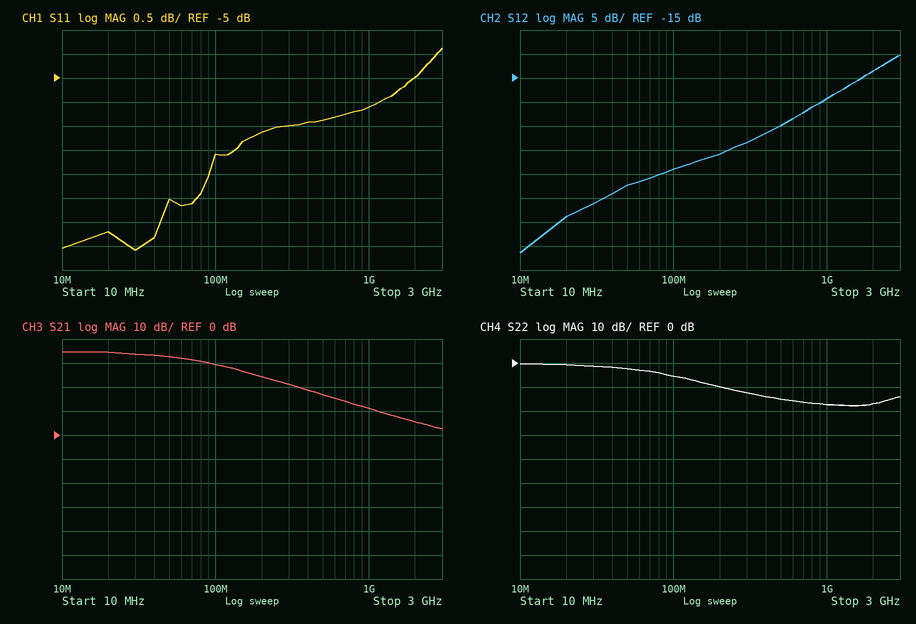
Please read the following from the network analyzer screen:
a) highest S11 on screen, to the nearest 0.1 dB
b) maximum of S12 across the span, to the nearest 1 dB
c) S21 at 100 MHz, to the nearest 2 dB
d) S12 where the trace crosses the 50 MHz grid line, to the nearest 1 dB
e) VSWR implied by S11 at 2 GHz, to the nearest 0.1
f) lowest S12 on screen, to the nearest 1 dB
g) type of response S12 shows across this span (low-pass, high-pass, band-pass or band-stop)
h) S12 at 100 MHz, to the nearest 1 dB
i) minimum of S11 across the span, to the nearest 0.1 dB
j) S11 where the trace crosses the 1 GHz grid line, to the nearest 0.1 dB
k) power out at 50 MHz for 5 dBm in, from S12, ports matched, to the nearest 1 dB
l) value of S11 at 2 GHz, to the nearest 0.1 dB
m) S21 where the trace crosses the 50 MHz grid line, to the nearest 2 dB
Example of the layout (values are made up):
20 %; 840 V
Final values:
-4.4 dB; -10 dB; 30 dB; -37 dB; 3.6; -51 dB; high-pass; -34 dB; -8.6 dB; -5.6 dB; -32 dBm; -5.0 dB; 32 dB
